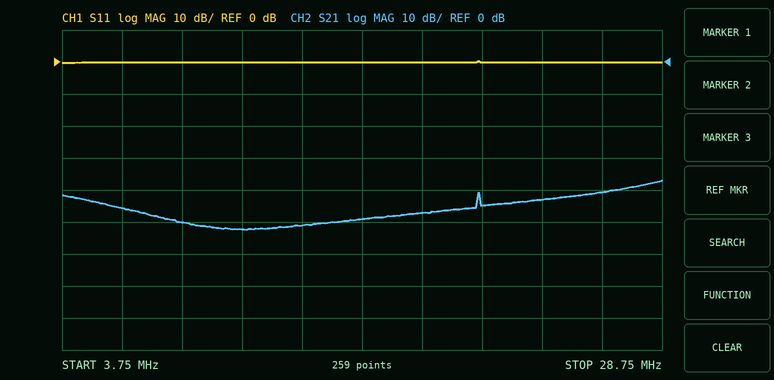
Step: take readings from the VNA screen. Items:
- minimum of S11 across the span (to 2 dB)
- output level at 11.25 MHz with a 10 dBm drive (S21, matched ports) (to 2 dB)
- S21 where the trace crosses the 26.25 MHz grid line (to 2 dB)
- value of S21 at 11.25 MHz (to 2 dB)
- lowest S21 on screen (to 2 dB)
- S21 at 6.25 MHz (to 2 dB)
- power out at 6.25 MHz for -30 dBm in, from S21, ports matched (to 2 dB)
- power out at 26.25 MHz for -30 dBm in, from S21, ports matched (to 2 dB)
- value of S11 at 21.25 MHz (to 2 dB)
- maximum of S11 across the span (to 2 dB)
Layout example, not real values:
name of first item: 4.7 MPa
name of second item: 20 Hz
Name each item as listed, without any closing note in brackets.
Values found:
minimum of S11 across the span: 0 dB
output level at 11.25 MHz with a 10 dBm drive (S21, matched ports): -42 dBm
S21 where the trace crosses the 26.25 MHz grid line: -40 dB
value of S21 at 11.25 MHz: -52 dB
lowest S21 on screen: -52 dB
S21 at 6.25 MHz: -46 dB
power out at 6.25 MHz for -30 dBm in, from S21, ports matched: -76 dBm
power out at 26.25 MHz for -30 dBm in, from S21, ports matched: -70 dBm
value of S11 at 21.25 MHz: 0 dB
maximum of S11 across the span: 0 dB
